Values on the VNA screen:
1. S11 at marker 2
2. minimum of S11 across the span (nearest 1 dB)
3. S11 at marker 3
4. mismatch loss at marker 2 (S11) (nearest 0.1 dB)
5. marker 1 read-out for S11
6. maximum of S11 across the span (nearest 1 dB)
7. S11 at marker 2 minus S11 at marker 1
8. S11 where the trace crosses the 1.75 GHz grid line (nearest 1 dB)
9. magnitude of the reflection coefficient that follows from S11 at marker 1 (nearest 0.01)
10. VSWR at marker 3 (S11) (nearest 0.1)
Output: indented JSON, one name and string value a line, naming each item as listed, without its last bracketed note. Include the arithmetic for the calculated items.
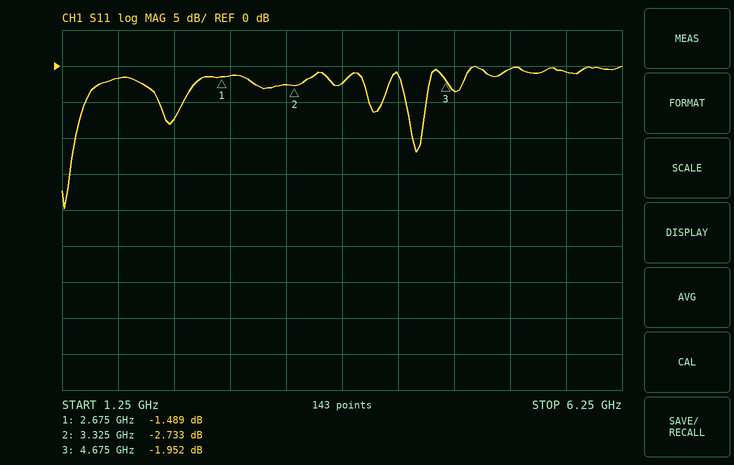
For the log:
{
  "S11 at marker 2": "-2.733 dB",
  "minimum of S11 across the span": "-20 dB",
  "S11 at marker 3": "-1.952 dB",
  "mismatch loss at marker 2 (S11)": "−10 log10(1 − 10^(-2.733/10)) ≈ 3.3 dB",
  "marker 1 read-out for S11": "-1.489 dB",
  "maximum of S11 across the span": "0 dB",
  "S11 at marker 2 minus S11 at marker 1": "-2.733 − (-1.489) = -1.244 dB",
  "S11 where the trace crosses the 1.75 GHz grid line": "-2 dB",
  "magnitude of the reflection coefficient that follows from S11 at marker 1": "10^(-1.489/20) ≈ 0.84",
  "VSWR at marker 3 (S11)": "(1 + 0.7987)/(1 − 0.7987) ≈ 8.9"
}
